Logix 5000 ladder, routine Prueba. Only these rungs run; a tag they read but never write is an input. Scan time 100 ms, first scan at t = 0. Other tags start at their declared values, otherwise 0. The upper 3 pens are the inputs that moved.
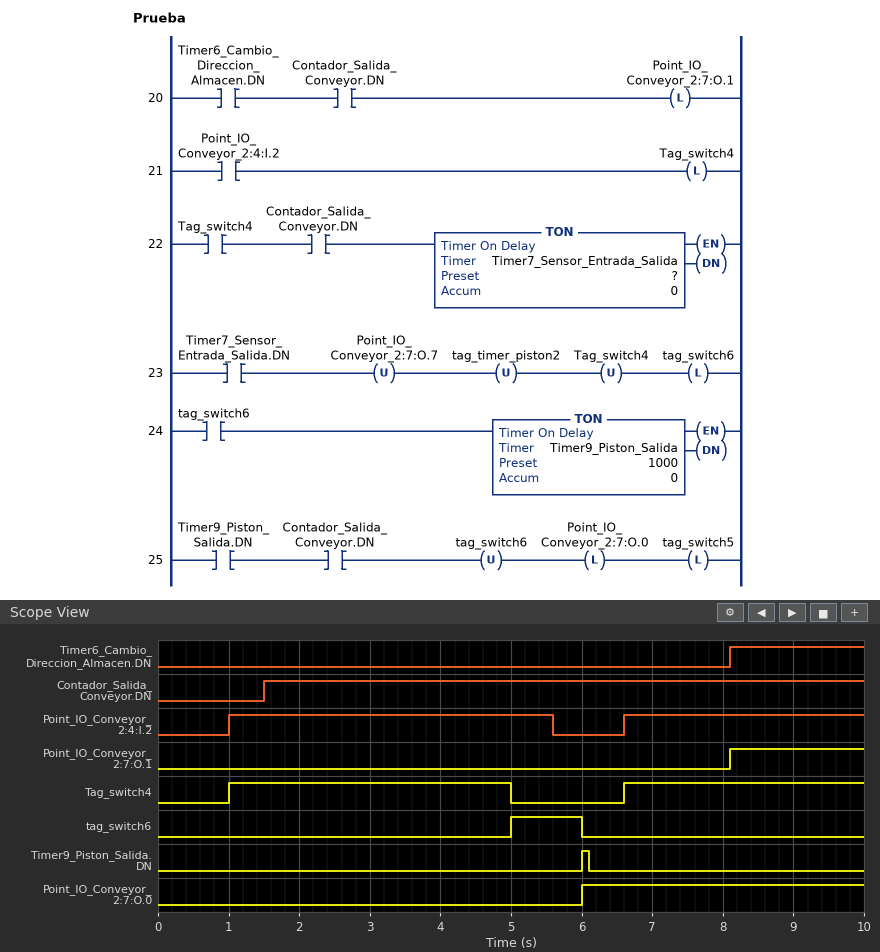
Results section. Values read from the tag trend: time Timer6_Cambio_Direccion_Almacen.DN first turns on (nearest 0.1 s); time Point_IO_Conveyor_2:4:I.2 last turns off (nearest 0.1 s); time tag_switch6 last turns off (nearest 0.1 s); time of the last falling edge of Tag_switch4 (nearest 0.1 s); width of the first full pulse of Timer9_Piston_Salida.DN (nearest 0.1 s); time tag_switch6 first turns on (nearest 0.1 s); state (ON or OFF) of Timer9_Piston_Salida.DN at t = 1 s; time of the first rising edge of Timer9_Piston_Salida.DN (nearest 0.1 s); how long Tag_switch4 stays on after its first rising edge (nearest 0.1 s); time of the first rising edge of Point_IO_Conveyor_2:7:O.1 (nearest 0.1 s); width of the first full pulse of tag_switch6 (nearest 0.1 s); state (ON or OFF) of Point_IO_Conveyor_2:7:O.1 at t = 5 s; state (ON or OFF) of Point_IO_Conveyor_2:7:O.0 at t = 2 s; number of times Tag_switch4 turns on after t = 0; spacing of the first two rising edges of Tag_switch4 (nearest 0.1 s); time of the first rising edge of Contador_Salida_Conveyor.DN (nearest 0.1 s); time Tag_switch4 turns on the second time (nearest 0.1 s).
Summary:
8.1 s
5.6 s
6.0 s
5.0 s
0.1 s
5.0 s
OFF
6.0 s
4.0 s
8.1 s
1.0 s
OFF
OFF
2
5.6 s
1.5 s
6.6 s
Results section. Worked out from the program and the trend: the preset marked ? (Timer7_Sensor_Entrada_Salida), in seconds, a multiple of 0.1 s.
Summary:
3.5 s
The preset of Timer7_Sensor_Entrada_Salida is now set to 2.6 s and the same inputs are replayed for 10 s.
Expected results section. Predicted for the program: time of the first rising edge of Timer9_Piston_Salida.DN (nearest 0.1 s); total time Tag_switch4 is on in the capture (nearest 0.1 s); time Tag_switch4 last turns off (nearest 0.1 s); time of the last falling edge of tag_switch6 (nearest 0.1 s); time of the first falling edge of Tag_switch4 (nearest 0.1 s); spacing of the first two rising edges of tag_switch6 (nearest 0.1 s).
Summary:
5.1 s
5.7 s
9.2 s
5.1 s
4.1 s
5.1 s
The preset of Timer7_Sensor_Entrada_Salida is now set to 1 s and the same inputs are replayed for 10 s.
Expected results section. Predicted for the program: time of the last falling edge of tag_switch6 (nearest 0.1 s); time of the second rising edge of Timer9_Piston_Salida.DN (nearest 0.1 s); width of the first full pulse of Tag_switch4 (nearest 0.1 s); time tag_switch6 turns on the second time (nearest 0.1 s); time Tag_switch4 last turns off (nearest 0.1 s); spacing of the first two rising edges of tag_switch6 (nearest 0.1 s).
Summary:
8.6 s
8.6 s
1.5 s
7.6 s
7.6 s
5.1 s
